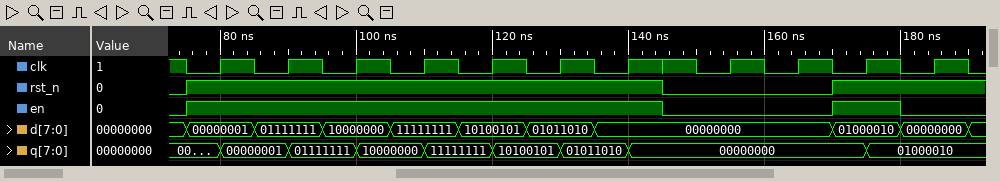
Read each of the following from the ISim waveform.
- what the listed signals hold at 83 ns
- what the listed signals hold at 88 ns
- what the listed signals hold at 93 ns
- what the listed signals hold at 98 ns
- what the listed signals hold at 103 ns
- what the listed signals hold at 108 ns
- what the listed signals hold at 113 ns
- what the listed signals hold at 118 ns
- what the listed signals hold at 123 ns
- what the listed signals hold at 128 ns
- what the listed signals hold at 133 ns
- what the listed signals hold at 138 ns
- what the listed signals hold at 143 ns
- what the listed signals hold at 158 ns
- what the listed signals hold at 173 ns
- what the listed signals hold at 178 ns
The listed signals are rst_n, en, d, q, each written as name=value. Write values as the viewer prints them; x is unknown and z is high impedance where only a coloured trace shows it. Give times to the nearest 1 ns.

rst_n=1, en=1, d=00000001, q=00000001
rst_n=1, en=1, d=01111111, q=00000001
rst_n=1, en=1, d=01111111, q=01111111
rst_n=1, en=1, d=10000000, q=01111111
rst_n=1, en=1, d=10000000, q=10000000
rst_n=1, en=1, d=11111111, q=10000000
rst_n=1, en=1, d=11111111, q=11111111
rst_n=1, en=1, d=10100101, q=11111111
rst_n=1, en=1, d=10100101, q=10100101
rst_n=1, en=1, d=01011010, q=10100101
rst_n=1, en=1, d=01011010, q=01011010
rst_n=1, en=1, d=00000000, q=01011010
rst_n=1, en=1, d=00000000, q=00000000
rst_n=0, en=0, d=00000000, q=00000000
rst_n=1, en=1, d=01000010, q=00000000
rst_n=1, en=1, d=01000010, q=01000010
